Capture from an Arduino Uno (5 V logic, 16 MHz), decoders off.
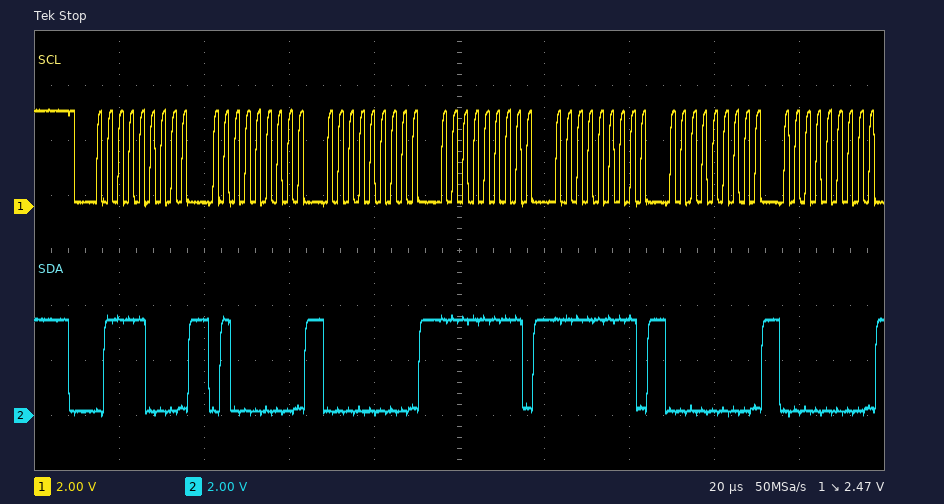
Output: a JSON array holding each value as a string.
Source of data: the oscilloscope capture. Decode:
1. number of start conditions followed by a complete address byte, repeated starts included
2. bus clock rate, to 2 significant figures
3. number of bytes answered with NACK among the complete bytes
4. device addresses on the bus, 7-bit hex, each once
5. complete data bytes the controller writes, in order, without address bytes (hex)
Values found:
["1", "400 kHz", "0", "0x3C", "40 00 FF FF 00 00"]
